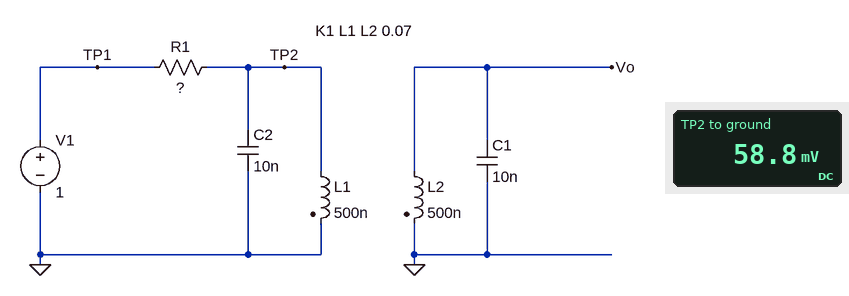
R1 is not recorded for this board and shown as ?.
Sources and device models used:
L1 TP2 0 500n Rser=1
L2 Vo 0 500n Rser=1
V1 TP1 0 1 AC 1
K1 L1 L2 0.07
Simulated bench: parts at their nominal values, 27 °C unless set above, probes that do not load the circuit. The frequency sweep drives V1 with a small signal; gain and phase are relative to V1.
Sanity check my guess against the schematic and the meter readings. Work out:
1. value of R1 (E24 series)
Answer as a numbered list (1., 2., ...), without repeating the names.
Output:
1. 16 Ω
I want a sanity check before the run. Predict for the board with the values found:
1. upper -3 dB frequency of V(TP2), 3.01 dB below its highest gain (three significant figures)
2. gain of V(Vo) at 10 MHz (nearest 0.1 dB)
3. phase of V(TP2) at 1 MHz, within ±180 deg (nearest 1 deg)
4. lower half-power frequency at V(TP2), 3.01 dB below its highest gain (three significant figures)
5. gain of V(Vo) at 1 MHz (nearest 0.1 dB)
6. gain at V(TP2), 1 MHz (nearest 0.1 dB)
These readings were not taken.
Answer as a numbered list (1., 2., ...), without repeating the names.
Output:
1. 3.14 MHz
2. -68.2 dB
3. 56 deg
4. 1.70 MHz
5. -34.5 dB
6. -12.8 dB
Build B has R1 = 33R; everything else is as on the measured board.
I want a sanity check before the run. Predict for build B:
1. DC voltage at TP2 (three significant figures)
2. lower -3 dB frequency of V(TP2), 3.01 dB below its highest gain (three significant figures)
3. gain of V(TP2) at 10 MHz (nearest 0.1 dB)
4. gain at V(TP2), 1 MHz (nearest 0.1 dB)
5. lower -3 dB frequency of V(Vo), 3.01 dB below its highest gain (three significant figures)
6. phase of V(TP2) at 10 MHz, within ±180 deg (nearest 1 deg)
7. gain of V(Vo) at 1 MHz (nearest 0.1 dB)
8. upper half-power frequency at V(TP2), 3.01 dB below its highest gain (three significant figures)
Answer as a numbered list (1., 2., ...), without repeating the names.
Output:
1. 29.4 mV
2. 1.85 MHz
3. -25.9 dB
4. -18.6 dB
5. 2.09 MHz
6. -87 deg
7. -40.2 dB
8. 2.80 MHz
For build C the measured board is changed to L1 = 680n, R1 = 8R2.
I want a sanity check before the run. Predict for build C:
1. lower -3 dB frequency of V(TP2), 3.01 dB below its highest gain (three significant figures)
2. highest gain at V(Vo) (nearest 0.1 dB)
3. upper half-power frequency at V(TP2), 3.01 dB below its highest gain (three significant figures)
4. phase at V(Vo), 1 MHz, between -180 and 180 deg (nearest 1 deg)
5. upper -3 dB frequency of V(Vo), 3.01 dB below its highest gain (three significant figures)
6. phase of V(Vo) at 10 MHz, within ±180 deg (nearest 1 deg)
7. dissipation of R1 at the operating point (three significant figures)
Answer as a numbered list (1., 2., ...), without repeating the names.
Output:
1. 1.21 MHz
2. -8.8 dB
3. 3.41 MHz
4. 51 deg
5. 2.40 MHz
6. 105 deg
7. 96.9 mW
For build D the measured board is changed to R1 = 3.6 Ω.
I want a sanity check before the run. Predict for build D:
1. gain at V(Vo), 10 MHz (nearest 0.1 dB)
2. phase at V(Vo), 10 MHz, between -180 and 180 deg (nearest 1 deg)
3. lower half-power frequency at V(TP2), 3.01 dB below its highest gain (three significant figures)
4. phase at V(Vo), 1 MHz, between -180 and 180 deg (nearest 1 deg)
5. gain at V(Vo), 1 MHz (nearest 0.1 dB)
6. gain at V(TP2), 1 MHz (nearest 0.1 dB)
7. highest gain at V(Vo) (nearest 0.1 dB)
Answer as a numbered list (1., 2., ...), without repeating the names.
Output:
1. -56.0 dB
2. 119 deg
3. 1.05 MHz
4. 45 deg
5. -25.5 dB
6. -3.9 dB
7. -7.0 dB
